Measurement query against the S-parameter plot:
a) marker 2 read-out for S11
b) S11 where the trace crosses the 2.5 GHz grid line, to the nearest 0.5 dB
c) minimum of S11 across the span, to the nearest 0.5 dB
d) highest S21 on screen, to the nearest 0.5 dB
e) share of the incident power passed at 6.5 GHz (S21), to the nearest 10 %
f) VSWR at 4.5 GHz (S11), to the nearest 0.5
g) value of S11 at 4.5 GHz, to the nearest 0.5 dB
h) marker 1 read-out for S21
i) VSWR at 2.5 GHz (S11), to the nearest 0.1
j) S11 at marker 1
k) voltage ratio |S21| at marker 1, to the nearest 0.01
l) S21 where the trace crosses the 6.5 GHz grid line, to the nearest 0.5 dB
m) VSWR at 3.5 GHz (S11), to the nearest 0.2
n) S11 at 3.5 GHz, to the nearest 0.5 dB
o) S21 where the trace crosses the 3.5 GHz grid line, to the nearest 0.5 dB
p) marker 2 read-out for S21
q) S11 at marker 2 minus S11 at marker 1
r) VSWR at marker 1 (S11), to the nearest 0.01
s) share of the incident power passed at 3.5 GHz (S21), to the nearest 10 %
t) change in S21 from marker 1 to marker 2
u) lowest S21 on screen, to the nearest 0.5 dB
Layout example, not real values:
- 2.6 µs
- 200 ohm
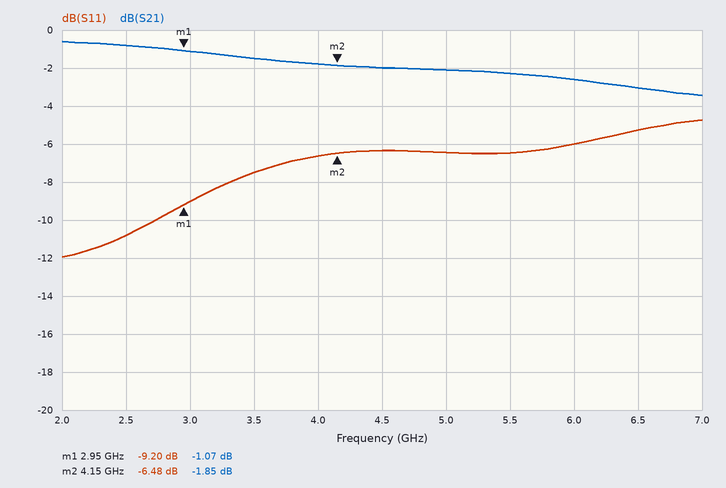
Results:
- -6.48 dB
- -11.0 dB
- -12.0 dB
- -0.5 dB
- 50 %
- 3.0
- -6.5 dB
- -1.07 dB
- 1.8
- -9.20 dB
- 0.88
- -3.0 dB
- 2.4
- -7.5 dB
- -1.5 dB
- -1.85 dB
- 2.72 dB
- 2.06
- 70 %
- -0.78 dB
- -3.5 dB
